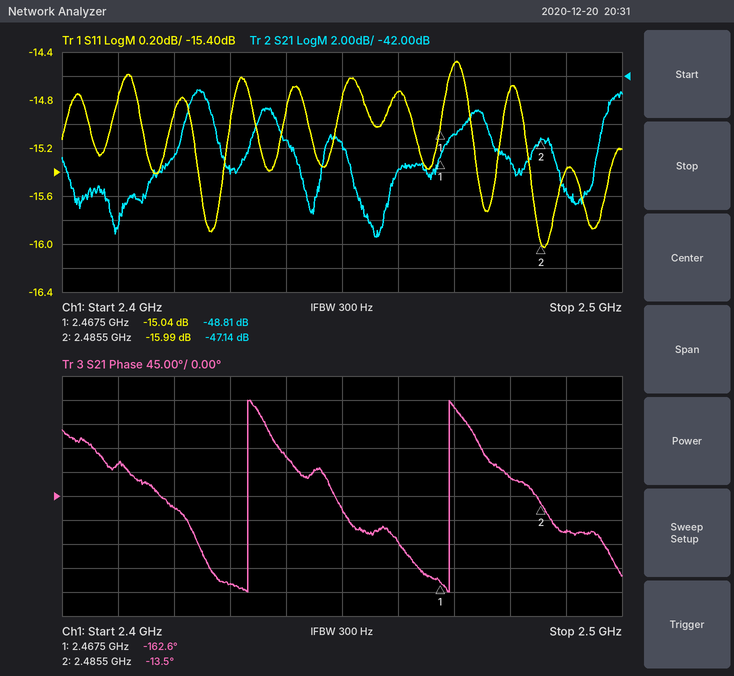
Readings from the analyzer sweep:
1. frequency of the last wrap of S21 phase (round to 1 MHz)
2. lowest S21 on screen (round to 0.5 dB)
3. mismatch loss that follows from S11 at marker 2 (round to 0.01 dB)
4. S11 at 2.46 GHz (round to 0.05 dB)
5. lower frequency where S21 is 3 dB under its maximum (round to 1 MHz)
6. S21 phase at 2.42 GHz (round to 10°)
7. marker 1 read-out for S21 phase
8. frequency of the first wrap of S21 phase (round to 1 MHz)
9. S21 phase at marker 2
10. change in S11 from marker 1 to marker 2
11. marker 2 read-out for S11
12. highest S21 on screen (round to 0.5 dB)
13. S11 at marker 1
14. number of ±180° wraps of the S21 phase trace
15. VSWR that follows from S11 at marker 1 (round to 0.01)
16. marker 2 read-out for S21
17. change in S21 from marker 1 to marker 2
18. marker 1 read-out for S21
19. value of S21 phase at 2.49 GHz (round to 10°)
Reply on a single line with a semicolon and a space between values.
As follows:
2.469 GHz; -55.5 dB; 0.11 dB; -14.75 dB; 2.422 GHz; -20°; -162.6°; 2.433 GHz; -13.5°; -0.95 dB; -15.99 dB; -43.0 dB; -15.04 dB; 2; 1.43; -47.14 dB; 1.67 dB; -48.81 dB; -70°
